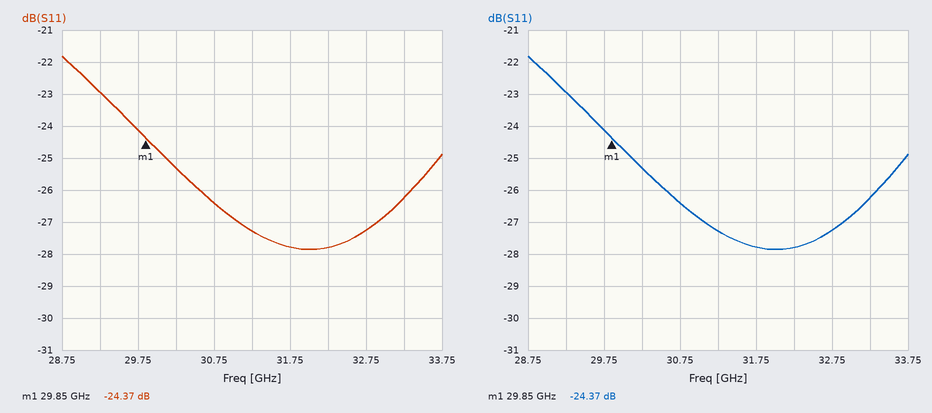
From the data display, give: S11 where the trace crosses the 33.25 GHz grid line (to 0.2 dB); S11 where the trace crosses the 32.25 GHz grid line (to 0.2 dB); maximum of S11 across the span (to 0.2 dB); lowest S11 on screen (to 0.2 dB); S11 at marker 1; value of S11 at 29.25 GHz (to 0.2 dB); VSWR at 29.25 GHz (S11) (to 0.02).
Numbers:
-26.2 dB
-27.8 dB
-21.8 dB
-27.8 dB
-24.37 dB
-23.0 dB
1.16
